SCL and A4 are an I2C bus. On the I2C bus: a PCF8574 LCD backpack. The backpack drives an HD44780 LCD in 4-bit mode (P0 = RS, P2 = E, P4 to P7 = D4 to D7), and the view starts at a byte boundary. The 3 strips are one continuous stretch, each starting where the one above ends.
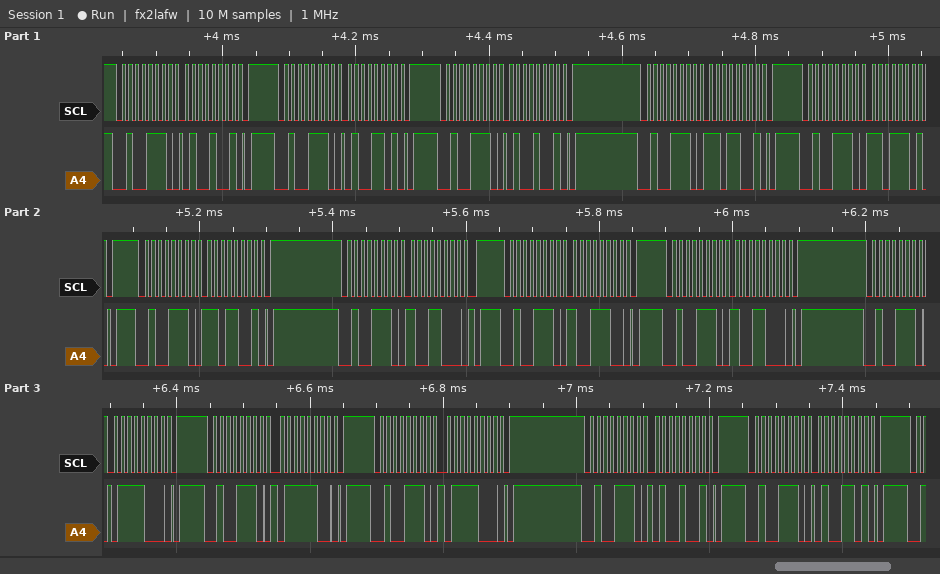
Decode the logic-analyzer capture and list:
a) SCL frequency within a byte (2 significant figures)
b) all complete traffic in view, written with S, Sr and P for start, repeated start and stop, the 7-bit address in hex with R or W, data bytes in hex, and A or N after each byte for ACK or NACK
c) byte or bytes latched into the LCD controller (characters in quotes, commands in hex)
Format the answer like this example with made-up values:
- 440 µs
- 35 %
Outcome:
- 100 kHz
- S 27W A 49 A P S 27W A 4D A P S 27W A 49 A P S 27W A D9 A P S 27W A DD A P S 27W A D9 A P S 27W A 98 A P S 27W A 9C A P S 27W A 98 A P S 27W A 78 A P S 27W A 7C A P S 27W A 78 A P S 27W A 49 A P S 27W A 4D A P
- 'M' 0x97
